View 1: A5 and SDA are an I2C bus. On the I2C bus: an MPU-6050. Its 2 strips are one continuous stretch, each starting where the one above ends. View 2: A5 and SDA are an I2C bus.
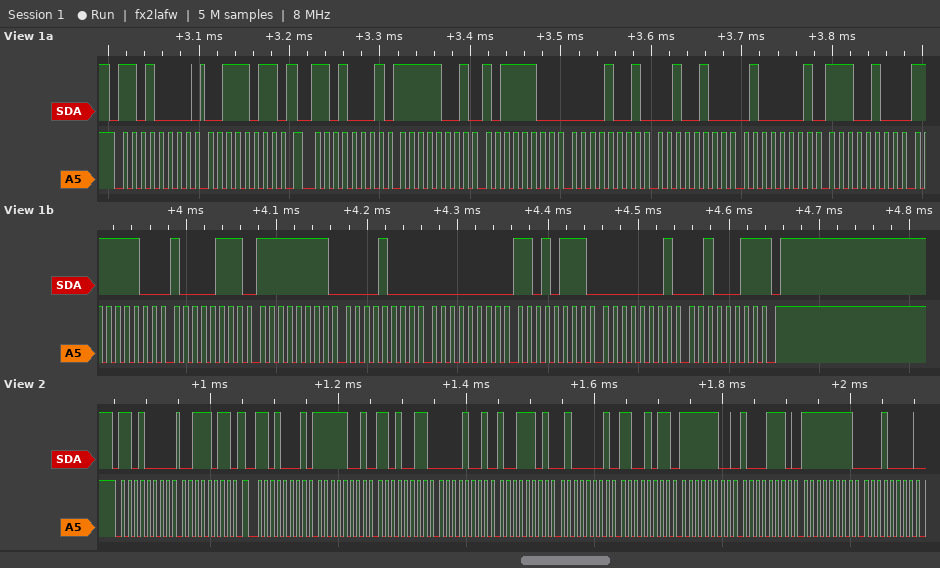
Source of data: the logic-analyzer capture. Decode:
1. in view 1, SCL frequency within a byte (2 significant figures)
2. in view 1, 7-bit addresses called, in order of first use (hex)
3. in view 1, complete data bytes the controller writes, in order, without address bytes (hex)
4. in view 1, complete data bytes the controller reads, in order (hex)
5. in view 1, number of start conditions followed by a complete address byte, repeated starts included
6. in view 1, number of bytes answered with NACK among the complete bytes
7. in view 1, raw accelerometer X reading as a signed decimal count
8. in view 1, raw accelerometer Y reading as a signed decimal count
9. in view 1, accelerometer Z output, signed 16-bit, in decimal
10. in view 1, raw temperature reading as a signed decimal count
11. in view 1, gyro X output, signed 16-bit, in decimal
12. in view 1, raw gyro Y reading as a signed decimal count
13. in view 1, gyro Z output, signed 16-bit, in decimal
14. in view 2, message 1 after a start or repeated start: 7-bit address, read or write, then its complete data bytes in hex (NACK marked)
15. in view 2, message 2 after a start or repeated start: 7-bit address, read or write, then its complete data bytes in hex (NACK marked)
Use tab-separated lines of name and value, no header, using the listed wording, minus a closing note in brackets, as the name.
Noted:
in view 1, SCL frequency within a byte	100 kHz
in view 1, 7-bit addresses called, in order of first use	0x68
in view 1, complete data bytes the controller writes, in order, without address bytes	3B
in view 1, complete data bytes the controller reads, in order	F9 BC 09 24 41 E4 FC 87 FF 08 00 D7 01 23
in view 1, number of start conditions followed by a complete address byte, repeated starts included	2
in view 1, number of bytes answered with NACK among the complete bytes	1
in view 1, raw accelerometer X reading as a signed decimal count	-1604
in view 1, raw accelerometer Y reading as a signed decimal count	2340
in view 1, accelerometer Z output, signed 16-bit, in decimal	16868
in view 1, raw temperature reading as a signed decimal count	-889
in view 1, gyro X output, signed 16-bit, in decimal	-248
in view 1, raw gyro Y reading as a signed decimal count	215
in view 1, gyro Z output, signed 16-bit, in decimal	291
in view 2, message 1 after a start or repeated start: 7-bit address, read or write, then its complete data bytes in hex	0x68 write: 3B
in view 2, message 2 after a start or repeated start: 7-bit address, read or write, then its complete data bytes in hex	0x68 read: F9 D3 09 9D 41 CB FC 8E FF 10
